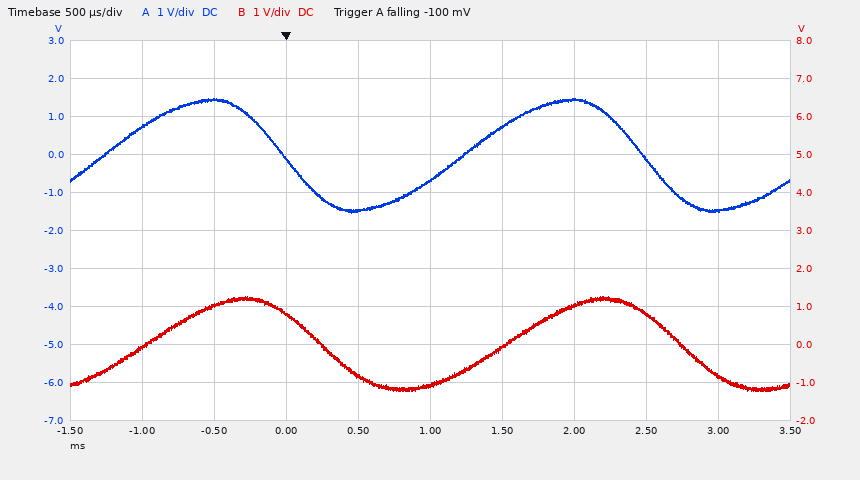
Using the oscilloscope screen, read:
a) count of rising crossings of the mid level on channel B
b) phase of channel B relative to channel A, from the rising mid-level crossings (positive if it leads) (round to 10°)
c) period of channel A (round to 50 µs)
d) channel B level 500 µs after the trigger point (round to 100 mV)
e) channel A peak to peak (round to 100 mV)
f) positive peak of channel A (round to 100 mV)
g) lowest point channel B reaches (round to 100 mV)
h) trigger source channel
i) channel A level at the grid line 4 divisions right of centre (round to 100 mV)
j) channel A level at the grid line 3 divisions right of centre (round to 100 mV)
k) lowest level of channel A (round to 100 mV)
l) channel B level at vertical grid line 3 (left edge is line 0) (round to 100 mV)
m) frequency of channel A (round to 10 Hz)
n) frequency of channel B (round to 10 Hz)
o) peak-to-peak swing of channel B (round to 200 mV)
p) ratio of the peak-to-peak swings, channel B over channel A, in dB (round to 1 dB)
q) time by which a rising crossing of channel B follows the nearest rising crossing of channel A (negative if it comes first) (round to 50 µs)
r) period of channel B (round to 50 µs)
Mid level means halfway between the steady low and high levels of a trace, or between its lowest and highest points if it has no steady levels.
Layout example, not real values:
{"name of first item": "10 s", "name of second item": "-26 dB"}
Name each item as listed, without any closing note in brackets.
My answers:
{"count of rising crossings of the mid level on channel B": "2", "phase of channel B relative to channel A, from the rising mid-level crossings (positive if it leads)": "-40°", "period of channel A": "2.50 ms", "channel B level 500 µs after the trigger point": "-800 mV", "channel A peak to peak": "3.0 V", "positive peak of channel A": "1.5 V", "lowest point channel B reaches": "-1.2 V", "trigger source channel": "channel A", "channel A level at the grid line 4 divisions right of centre": "-1.5 V", "channel A level at the grid line 3 divisions right of centre": "-100 mV", "lowest level of channel A": "-1.5 V", "channel B level at vertical grid line 3 (left edge is line 0)": "800 mV", "frequency of channel A": "400 Hz", "frequency of channel B": "400 Hz", "peak-to-peak swing of channel B": "2.4 V", "ratio of the peak-to-peak swings, channel B over channel A, in dB": "-2 dB", "time by which a rising crossing of channel B follows the nearest rising crossing of channel A (negative if it comes first)": "+300 µs", "period of channel B": "2.50 ms"}
